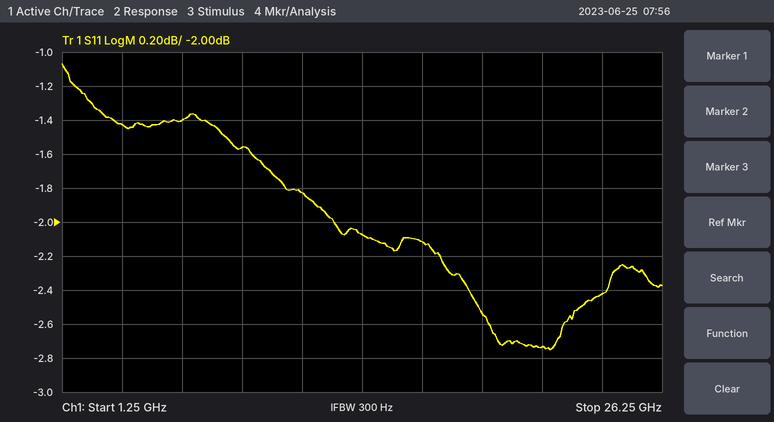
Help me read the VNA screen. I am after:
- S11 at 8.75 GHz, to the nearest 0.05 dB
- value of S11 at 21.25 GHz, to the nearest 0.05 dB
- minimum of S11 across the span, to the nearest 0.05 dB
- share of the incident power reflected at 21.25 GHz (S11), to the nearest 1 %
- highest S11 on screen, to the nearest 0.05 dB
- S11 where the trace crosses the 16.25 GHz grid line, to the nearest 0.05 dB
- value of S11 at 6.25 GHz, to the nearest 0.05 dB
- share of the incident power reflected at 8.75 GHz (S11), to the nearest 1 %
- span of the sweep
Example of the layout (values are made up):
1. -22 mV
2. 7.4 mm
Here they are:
1. -1.55 dB
2. -2.75 dB
3. -2.75 dB
4. 53 %
5. -1.05 dB
6. -2.10 dB
7. -1.40 dB
8. 70 %
9. 25 GHz
